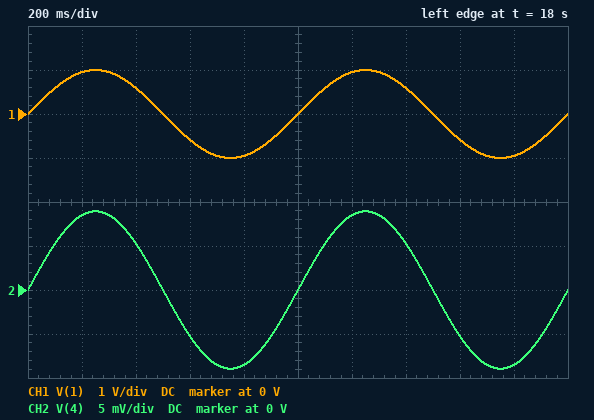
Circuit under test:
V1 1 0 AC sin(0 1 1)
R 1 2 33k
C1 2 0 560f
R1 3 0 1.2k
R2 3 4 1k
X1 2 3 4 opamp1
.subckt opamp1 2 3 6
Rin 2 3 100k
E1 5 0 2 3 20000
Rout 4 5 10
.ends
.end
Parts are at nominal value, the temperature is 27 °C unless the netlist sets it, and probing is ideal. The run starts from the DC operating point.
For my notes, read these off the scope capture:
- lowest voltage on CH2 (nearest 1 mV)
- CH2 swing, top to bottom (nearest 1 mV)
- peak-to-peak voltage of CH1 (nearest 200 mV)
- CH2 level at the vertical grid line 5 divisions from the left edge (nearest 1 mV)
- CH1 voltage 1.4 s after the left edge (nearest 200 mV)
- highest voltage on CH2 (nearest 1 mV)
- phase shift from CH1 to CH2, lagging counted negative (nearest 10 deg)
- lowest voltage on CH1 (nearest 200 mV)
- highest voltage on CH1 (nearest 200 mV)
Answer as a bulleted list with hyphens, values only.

- -9 mV
- 18 mV
- 2.0 V
- 0 V
- 600 mV
- 9 mV
- 0 deg
- -1.0 V
- 1.0 V
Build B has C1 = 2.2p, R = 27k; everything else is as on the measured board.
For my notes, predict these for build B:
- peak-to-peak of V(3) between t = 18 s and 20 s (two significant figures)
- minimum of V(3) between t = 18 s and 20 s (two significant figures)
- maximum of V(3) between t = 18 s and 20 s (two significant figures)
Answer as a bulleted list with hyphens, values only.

- 19 mV
- -9.4 mV
- 9.4 mV
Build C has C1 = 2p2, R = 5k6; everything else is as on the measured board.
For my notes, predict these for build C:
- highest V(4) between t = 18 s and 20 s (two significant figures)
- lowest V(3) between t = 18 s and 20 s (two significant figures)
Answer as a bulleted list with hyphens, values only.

- 11 mV
- -11 mV
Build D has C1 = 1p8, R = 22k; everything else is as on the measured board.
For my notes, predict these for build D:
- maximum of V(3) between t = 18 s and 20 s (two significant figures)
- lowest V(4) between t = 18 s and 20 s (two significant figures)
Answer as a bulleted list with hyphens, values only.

- 9.7 mV
- -9.7 mV
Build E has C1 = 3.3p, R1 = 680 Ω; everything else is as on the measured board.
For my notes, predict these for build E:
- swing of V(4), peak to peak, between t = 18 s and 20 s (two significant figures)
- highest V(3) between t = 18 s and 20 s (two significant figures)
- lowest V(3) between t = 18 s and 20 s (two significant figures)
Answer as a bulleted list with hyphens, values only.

- 10 mV
- 5.1 mV
- -5.1 mV
